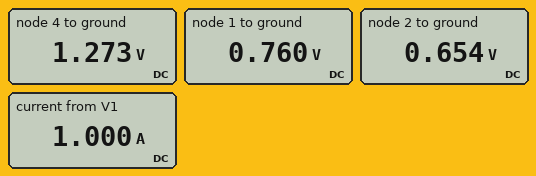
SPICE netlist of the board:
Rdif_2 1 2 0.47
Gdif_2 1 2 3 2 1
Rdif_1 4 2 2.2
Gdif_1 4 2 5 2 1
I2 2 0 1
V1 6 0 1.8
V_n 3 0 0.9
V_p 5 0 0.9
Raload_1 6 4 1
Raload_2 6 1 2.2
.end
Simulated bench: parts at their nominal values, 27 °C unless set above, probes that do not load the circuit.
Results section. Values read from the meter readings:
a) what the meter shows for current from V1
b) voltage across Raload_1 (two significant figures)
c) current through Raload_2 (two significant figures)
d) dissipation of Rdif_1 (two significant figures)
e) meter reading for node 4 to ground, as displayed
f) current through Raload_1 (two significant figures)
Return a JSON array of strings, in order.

["1.000 A", "530 mV", "470 mA", "170 mW", "1.273 V", "530 mA"]
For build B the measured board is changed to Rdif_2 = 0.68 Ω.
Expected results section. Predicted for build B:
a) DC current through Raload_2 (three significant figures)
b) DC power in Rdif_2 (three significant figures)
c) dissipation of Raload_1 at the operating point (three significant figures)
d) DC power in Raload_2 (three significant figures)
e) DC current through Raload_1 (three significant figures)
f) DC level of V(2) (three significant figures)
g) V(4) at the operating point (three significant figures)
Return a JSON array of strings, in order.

["462 mA", "28.7 mW", "289 mW", "470 mW", "538 mA", "643 mV", "1.26 V"]
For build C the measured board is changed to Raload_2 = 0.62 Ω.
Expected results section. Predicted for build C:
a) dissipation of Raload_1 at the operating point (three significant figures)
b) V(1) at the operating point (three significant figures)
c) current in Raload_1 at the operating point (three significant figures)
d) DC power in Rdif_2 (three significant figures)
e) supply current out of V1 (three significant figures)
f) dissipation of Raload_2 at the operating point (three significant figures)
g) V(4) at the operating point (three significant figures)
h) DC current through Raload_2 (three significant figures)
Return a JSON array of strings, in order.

["55.6 mW", "1.33 V", "236 mA", "308 mW", "1.00 A", "362 mW", "1.56 V", "764 mA"]
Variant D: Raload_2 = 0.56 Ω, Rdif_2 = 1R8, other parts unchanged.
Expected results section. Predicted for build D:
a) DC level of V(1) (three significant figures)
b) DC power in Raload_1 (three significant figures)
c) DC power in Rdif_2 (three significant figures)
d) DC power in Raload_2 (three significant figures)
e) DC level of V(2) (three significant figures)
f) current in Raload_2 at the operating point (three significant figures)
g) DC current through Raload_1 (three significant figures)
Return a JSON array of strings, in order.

["1.48 V", "190 mW", "303 mW", "178 mW", "746 mV", "564 mA", "436 mA"]
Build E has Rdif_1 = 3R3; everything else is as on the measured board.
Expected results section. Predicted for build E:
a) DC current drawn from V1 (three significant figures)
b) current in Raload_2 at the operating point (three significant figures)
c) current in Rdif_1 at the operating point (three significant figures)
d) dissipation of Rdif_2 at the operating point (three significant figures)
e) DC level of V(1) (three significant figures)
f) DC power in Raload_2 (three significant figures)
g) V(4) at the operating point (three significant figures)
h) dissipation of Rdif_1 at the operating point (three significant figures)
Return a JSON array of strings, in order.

["1.00 A", "498 mA", "209 mA", "19.9 mW", "704 mV", "546 mW", "1.30 V", "145 mW"]
